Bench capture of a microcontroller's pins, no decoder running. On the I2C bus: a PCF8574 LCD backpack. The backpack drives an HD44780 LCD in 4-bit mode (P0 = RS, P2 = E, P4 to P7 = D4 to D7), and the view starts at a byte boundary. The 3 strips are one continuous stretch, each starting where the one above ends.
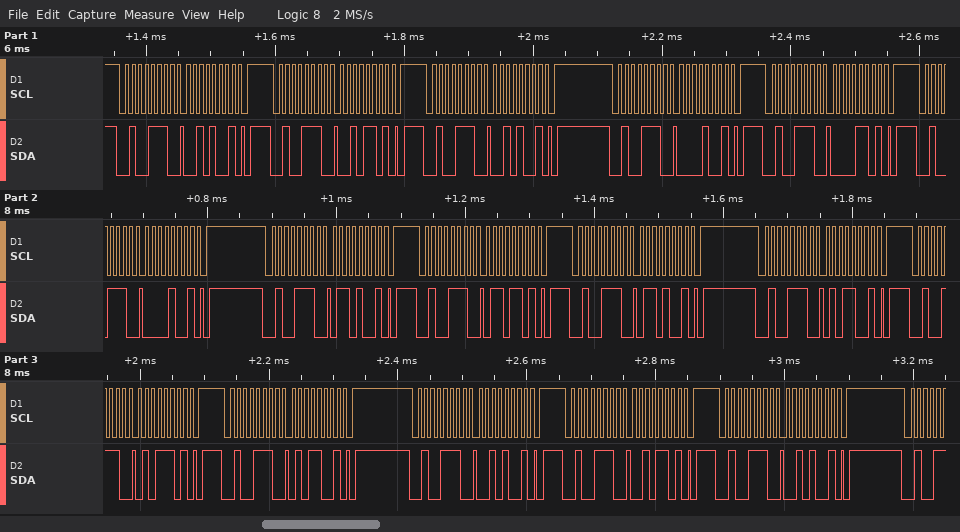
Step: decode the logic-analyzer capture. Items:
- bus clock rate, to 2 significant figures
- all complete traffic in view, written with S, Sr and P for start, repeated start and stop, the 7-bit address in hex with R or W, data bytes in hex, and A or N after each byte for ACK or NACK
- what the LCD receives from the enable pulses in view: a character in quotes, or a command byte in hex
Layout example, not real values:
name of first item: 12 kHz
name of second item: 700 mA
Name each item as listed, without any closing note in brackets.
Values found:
bus clock rate, to 2 significant figures: 100 kHz
all complete traffic in view, written with S, Sr and P for start, repeated start and stop, the 7-bit address in hex with R or W, data bytes in hex, and A or N after each byte for ACK or NACK: S 27W A 29 A P S 27W A 2D A P S 27W A 29 A P S 27W A 09 A P S 27W A 0D A P S 27W A 09 A P S 27W A 69 A P S 27W A 6D A P S 27W A 69 A P S 27W A 59 A P S 27W A 5D A P S 27W A 59 A P S 27W A 29 A P S 27W A 2D A P S 27W A 29 A P
what the LCD receives from the enable pulses in view: a character in quotes, or a command byte in hex: ' ' 'e'
